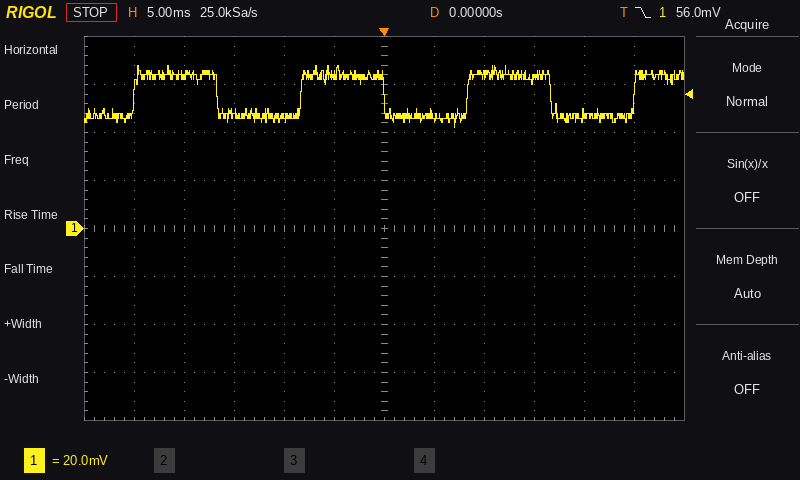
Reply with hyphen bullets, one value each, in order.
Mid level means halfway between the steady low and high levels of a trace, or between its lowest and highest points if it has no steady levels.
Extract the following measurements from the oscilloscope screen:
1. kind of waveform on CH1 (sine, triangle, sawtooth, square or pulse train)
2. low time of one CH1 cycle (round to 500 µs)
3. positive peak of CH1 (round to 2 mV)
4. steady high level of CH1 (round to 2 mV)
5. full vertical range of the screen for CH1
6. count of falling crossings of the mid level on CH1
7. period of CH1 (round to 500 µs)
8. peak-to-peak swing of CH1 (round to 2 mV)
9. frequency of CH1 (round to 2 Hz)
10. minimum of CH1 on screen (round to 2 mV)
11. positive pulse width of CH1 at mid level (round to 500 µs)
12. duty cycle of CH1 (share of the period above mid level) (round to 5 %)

- square
- 8.5 ms
- 68 mV
- 64 mV
- 160 mV
- 3
- 16.5 ms
- 26 mV
- 60 Hz
- 42 mV
- 8.5 ms
- 50 %
